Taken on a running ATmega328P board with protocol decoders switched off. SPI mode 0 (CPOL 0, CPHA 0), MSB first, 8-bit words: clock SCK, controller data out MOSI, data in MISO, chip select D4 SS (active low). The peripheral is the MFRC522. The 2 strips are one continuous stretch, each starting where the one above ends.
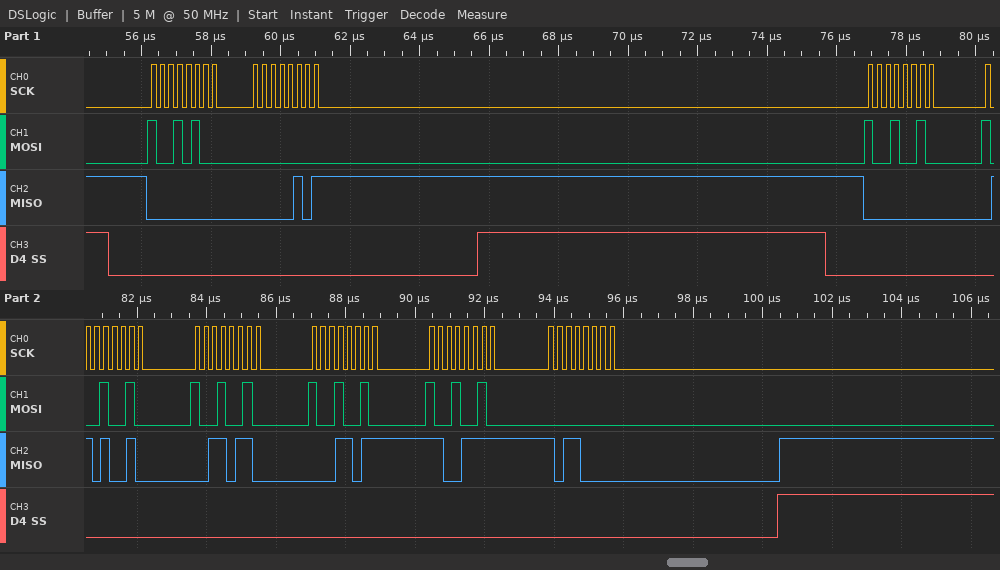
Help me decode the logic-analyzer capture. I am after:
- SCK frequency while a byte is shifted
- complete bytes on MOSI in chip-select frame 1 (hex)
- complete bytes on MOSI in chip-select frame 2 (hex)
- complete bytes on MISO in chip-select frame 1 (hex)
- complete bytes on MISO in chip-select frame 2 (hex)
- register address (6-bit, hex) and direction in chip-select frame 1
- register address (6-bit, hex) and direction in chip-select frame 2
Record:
4 MHz
0x94 0x00
0x92 0x92 0x92 0x92 0x92 0x00
0x00 0x05
0x00 0x52 0x36 0x1B 0xCF 0xB0
0x0A read
0x09 read
